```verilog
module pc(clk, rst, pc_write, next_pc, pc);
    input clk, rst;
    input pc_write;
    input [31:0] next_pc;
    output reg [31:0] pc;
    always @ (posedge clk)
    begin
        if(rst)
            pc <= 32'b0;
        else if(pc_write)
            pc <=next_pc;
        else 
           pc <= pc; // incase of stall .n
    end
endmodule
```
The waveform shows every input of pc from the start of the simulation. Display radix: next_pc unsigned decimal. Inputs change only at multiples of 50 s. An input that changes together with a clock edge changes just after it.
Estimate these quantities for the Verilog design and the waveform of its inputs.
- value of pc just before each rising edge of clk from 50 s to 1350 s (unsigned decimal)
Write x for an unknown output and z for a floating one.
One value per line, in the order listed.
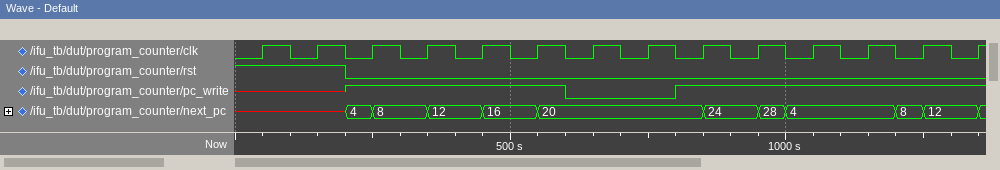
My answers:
x, 0, 0, 4, 8, 12, 16, 16, 16, 20, 24, 4, 4, 8
